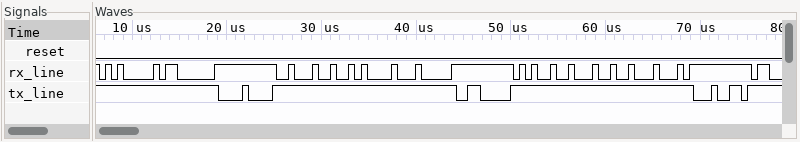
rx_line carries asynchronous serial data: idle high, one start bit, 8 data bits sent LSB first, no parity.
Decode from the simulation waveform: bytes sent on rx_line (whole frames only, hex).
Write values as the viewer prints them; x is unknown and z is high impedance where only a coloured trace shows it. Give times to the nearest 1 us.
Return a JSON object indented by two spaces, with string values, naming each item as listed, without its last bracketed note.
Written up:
{
  "bytes sent on rx_line": "05, 03, 22, 0A, 04, 25, 24, 44"
}
